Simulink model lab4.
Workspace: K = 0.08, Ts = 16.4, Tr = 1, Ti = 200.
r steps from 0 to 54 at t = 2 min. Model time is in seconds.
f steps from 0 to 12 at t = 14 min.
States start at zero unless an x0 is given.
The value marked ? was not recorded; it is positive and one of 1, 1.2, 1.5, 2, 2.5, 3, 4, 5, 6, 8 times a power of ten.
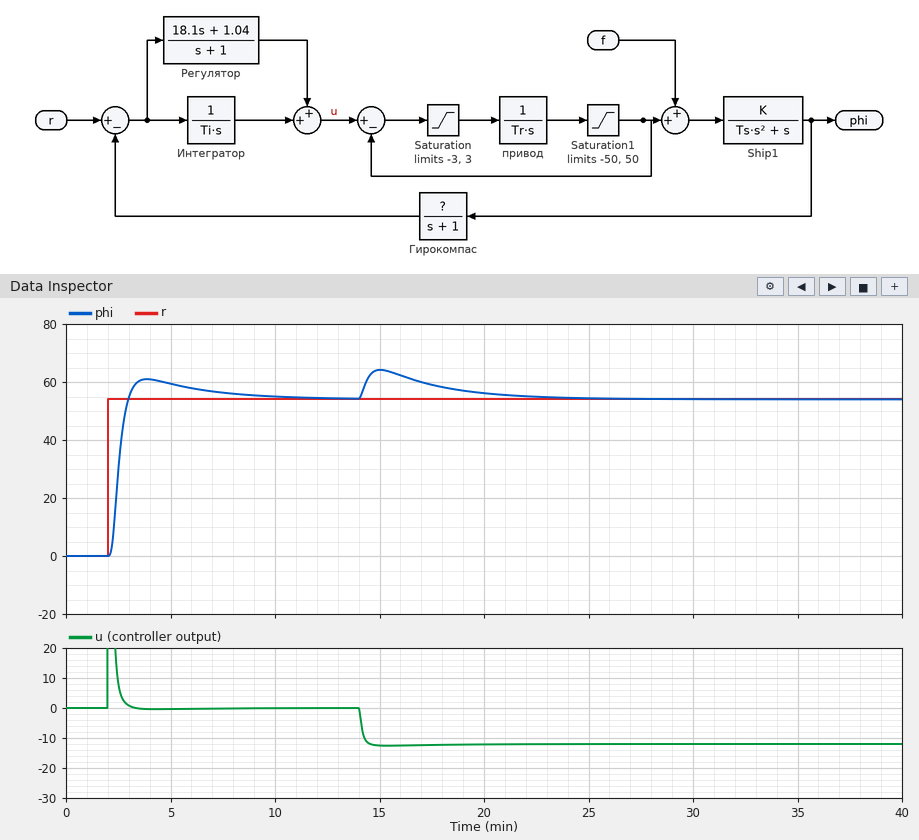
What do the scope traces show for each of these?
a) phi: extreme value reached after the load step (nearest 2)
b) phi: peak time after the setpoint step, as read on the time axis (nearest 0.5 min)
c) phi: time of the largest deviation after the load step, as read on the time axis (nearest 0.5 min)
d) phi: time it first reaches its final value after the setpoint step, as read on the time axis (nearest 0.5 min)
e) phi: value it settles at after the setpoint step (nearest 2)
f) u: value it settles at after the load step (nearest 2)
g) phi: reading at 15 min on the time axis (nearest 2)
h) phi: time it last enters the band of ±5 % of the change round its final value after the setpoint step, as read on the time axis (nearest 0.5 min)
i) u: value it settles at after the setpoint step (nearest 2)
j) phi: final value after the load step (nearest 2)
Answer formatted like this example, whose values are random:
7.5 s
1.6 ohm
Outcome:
64
4.0 min
15.0 min
3.0 min
54
-12
64
7.0 min
0
54
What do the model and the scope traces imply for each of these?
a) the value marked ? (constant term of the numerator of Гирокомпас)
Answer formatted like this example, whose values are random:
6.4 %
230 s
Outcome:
1
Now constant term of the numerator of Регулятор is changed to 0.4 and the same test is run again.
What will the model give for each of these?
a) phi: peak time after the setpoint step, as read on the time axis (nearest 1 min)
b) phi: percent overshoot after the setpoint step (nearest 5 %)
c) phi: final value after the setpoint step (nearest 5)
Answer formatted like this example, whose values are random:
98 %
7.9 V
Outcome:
5 min
35 %
55
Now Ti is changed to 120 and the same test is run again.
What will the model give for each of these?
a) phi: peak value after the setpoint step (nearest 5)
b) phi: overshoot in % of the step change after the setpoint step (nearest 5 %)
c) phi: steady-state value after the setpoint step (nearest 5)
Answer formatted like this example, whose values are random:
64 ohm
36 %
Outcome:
65
20 %
55
